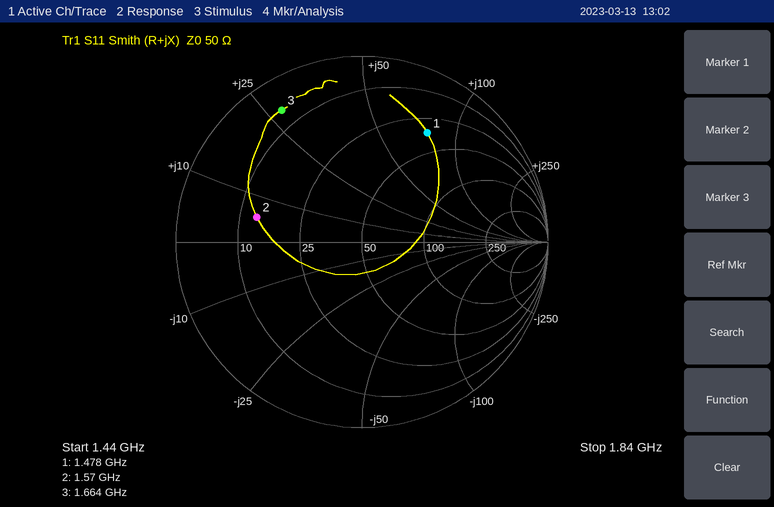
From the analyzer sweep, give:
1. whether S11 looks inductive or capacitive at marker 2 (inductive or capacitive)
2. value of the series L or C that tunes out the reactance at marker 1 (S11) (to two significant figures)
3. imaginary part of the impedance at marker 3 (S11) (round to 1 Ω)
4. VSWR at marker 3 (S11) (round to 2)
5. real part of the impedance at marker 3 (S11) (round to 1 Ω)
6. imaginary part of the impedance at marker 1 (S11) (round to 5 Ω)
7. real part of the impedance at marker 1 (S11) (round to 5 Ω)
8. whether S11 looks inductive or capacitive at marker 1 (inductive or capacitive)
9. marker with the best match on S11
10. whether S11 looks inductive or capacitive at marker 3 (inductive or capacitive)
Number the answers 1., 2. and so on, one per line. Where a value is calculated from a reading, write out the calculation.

1. inductive
2. C = 1/(2π × 1.478 GHz × 75 Ω) ≈ 1.4 pF
3. +28 Ω
4. 10
5. 6 Ω
6. +75 Ω
7. 35 Ω
8. inductive
9. marker 2
10. inductive
